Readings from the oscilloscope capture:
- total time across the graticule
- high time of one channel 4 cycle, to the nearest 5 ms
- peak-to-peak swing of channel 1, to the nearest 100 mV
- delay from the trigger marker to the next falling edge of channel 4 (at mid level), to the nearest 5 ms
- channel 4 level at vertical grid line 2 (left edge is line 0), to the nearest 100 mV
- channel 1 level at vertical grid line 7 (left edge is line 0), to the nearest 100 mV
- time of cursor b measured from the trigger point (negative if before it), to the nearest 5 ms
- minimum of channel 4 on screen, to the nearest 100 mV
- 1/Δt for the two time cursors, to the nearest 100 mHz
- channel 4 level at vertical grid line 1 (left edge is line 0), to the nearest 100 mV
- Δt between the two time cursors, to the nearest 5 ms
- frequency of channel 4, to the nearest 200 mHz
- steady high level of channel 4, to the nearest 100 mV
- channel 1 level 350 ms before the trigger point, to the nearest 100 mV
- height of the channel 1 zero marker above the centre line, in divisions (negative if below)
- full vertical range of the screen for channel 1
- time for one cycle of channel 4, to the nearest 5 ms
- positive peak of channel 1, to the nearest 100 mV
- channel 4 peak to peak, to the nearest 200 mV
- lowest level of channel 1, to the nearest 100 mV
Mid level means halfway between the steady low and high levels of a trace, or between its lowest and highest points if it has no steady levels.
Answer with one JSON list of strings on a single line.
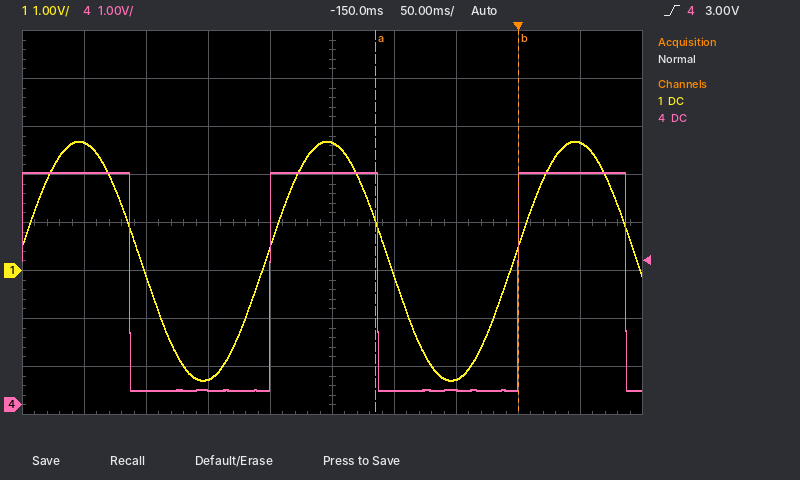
["500 ms", "85 ms", "5.0 V", "85 ms", "300 mV", "-2.3 V", "0 ms", "300 mV", "8.7 Hz", "4.8 V", "115 ms", "5.0 Hz", "4.8 V", "2.7 V", "-1.0 div", "8 V", "200 ms", "2.7 V", "4.6 V", "-2.3 V"]
